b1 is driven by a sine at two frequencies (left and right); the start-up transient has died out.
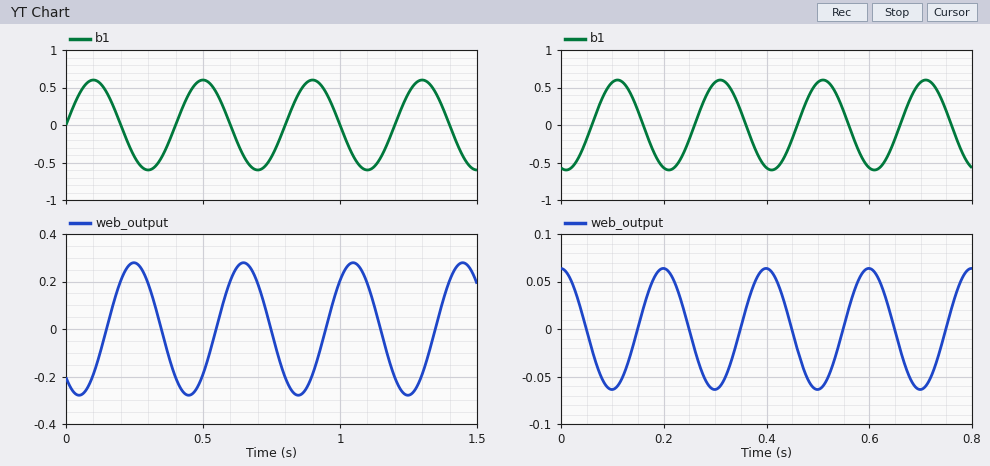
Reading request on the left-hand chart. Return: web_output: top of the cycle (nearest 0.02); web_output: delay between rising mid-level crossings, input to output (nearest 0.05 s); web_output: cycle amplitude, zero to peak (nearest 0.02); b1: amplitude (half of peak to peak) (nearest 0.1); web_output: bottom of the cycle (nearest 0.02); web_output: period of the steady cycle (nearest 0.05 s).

0.28
0.15 s
0.28
0.6
-0.28
0.40 s
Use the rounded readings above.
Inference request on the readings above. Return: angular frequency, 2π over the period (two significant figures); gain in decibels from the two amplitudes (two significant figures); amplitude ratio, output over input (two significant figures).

16 rad/s
-6.6 dB
0.47
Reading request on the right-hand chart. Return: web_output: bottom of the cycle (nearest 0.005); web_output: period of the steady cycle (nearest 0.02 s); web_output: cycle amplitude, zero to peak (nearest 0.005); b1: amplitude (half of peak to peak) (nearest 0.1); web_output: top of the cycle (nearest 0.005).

-0.065
0.20 s
0.065
0.6
0.065
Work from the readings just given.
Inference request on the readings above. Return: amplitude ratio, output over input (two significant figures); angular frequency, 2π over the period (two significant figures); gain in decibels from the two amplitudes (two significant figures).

0.11
31 rad/s
-19 dB
